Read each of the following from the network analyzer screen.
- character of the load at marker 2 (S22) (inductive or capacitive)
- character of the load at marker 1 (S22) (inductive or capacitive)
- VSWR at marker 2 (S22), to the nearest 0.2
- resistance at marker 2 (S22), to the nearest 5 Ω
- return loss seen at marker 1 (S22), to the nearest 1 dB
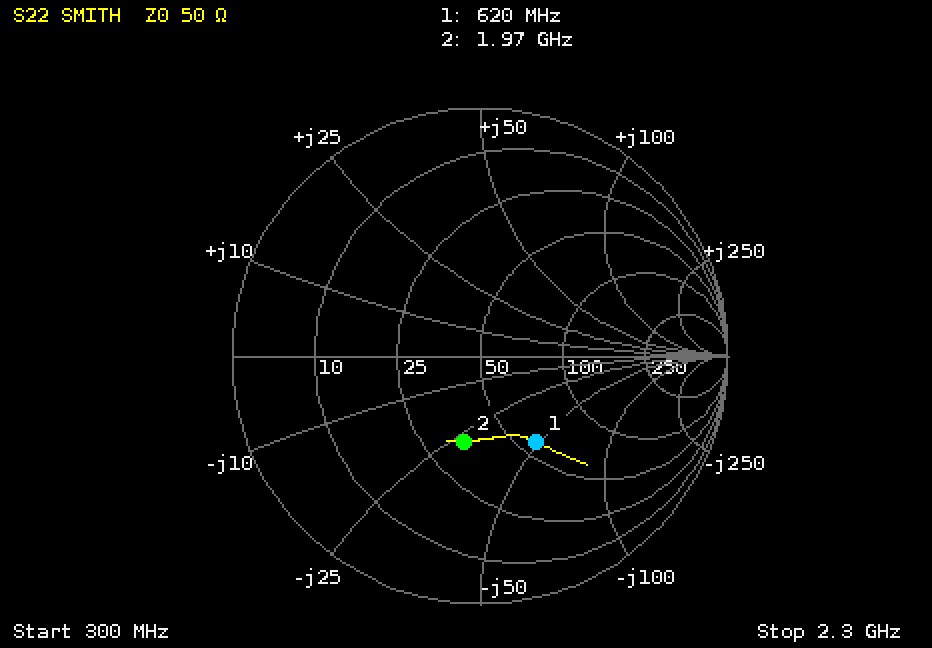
capacitive
capacitive
2.0
35 Ω
8 dB
